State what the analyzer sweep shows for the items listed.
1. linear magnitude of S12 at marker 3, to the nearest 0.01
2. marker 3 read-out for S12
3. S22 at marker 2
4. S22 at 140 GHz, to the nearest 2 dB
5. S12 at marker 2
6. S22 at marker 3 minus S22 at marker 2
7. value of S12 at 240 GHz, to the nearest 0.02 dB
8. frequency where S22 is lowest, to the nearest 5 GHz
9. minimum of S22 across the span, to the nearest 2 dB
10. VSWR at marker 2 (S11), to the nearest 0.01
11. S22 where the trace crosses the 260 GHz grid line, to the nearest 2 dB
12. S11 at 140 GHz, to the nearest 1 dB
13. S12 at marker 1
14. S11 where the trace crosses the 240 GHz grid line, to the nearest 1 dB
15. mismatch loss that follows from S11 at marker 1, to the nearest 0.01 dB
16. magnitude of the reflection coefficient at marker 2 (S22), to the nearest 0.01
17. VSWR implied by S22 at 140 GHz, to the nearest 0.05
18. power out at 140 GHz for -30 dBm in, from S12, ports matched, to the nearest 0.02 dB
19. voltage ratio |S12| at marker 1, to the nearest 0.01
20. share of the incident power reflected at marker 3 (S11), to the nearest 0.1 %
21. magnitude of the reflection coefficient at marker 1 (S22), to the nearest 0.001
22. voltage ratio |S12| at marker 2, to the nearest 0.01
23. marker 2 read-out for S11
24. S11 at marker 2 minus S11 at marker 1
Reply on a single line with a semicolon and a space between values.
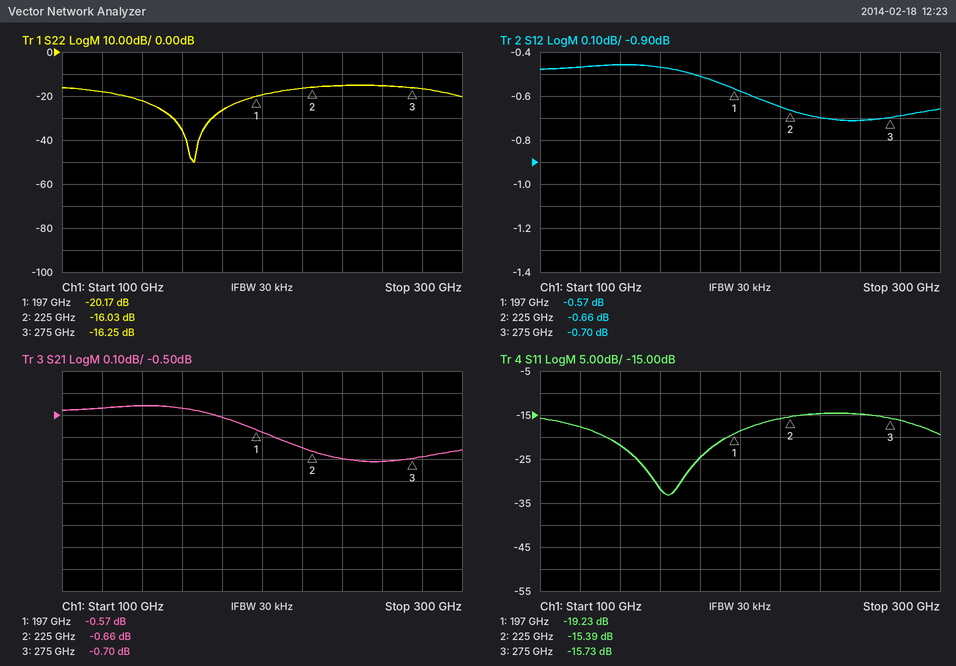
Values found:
0.92; -0.70 dB; -16.03 dB; -22 dB; -0.66 dB; -0.22 dB; -0.70 dB; 165 GHz; -50 dB; 1.41; -16 dB; -22 dB; -0.57 dB; -15 dB; 0.05 dB; 0.16; 1.15; -30.46 dBm; 0.94; 2.7 %; 0.098; 0.93; -15.39 dB; 3.84 dB
